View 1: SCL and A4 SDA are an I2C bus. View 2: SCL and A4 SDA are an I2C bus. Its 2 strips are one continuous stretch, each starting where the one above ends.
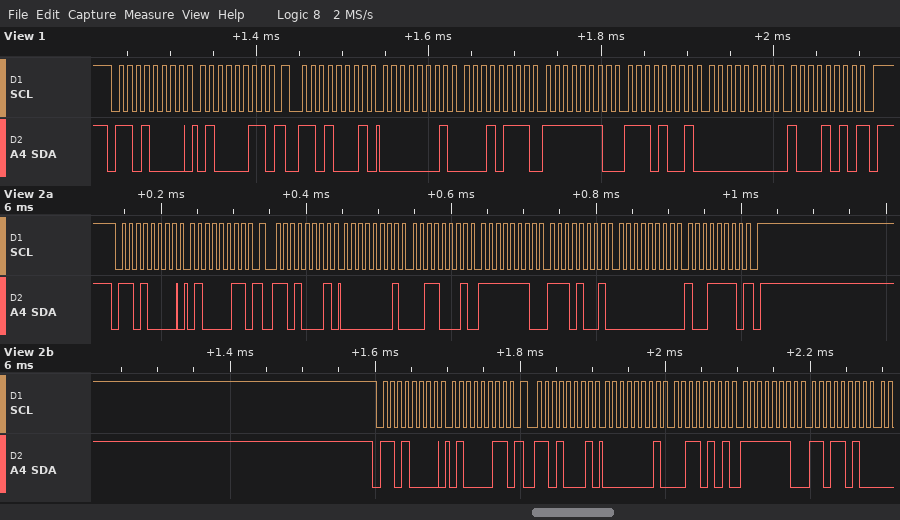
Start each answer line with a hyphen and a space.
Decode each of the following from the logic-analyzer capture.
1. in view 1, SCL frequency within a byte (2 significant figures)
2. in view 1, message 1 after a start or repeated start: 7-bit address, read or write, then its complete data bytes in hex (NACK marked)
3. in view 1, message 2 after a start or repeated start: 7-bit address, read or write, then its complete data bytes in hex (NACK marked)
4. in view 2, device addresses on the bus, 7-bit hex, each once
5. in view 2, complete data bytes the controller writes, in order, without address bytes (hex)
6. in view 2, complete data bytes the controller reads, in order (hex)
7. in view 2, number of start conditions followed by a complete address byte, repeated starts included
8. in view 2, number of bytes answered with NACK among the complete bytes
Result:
- 100 kHz
- 0x68 write: 43
- 0x68 read: 01 17 FE E9 00 8A NACK
- 0x68
- 43 43
- 01 31 FE E9 00 9E 01 35 FE DA
- 4
- 1
